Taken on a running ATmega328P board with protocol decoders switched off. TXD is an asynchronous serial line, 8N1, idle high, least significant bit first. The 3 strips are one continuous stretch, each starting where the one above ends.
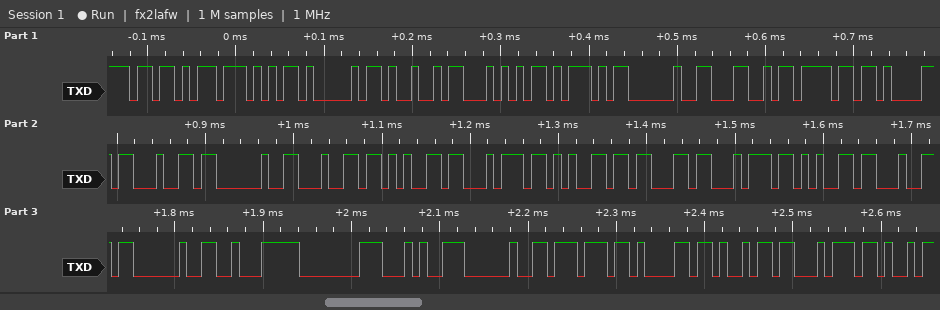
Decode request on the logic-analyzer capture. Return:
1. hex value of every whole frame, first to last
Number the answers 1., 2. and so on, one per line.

1. 5B 57 41 49 54 5D 20 4C 6F 61 64 20 64 65 74 65 63 74 65 64 20 E2 80 94 20 77 61 69 74
